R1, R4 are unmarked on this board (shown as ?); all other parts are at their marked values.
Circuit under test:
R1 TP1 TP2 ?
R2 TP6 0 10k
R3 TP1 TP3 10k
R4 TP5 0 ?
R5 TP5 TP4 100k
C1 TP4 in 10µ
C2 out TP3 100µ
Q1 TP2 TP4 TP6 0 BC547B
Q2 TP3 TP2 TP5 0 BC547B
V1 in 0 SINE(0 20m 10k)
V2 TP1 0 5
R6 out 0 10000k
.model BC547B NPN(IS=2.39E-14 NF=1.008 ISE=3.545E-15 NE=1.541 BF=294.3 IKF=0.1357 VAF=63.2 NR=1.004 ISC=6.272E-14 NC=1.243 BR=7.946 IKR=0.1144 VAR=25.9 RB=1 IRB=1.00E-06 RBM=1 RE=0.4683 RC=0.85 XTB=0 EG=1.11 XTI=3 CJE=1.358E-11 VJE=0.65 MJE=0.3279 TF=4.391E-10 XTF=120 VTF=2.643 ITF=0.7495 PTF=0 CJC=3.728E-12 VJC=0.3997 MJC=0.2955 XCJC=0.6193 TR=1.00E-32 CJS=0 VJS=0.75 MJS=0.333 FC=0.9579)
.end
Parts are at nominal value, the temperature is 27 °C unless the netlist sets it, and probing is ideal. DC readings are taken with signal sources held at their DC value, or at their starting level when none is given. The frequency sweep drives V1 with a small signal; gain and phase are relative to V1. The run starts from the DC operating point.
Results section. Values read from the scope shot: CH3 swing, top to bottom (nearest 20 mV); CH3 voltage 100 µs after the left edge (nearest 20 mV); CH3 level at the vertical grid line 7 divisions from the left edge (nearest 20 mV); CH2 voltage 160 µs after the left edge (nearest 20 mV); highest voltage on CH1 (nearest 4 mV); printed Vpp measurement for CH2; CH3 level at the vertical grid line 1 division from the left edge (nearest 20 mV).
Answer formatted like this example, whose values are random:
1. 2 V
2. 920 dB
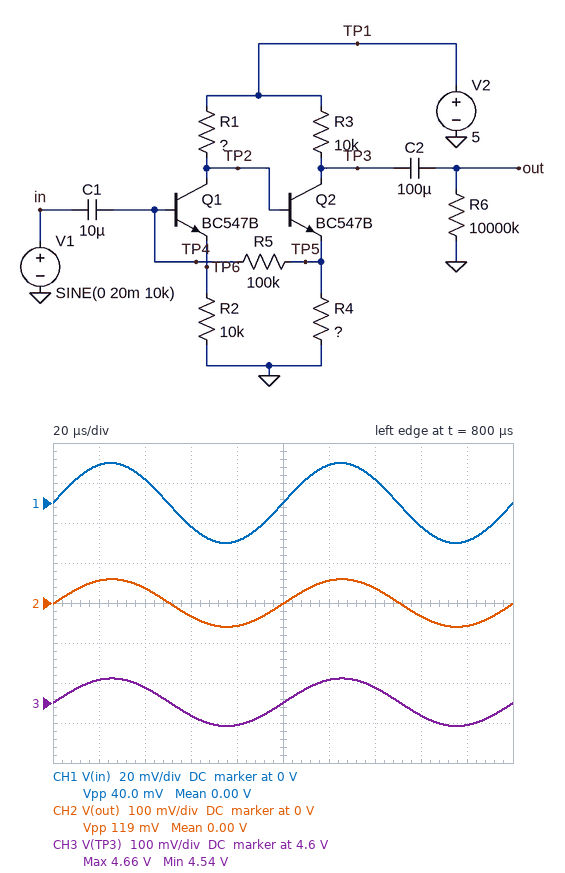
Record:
1. 120 mV
2. 4.60 V
3. 4.64 V
4. -40 mV
5. 20 mV
6. 119 mV
7. 4.66 V
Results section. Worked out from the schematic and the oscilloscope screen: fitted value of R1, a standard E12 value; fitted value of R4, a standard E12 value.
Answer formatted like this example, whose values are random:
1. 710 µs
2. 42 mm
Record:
1. 68 kΩ
2. 27 kΩ
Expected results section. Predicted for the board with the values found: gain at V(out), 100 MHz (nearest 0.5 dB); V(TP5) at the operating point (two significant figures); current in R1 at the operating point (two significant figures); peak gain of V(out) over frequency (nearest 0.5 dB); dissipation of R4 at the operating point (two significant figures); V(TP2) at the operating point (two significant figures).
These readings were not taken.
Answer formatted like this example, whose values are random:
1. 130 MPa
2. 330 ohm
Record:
1. 0 dB
2. 1.1 V
3. 50 µA
4. 9.5 dB
5. 43 µW
6. 1.6 V
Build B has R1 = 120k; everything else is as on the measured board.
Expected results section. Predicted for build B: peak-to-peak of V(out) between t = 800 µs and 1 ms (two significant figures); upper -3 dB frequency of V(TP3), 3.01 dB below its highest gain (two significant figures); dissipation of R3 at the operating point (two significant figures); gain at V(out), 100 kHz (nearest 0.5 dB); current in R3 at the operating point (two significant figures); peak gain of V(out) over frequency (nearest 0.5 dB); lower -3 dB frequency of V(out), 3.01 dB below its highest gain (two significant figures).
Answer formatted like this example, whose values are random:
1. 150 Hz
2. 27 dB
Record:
1. 200 mV
2. 200 kHz
3. 10 µW
4. 13.0 dB
5. 32 µA
6. 14.0 dB
7. 1.8 Hz
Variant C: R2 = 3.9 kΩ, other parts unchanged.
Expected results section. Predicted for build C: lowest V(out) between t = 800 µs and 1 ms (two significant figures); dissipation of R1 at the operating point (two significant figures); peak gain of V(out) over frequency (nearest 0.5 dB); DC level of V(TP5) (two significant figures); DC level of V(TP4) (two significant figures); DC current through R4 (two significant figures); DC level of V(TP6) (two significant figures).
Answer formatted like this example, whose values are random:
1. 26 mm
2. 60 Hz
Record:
1. -140 mV
2. 200 µW
3. 17.0 dB
4. 790 mV
5. 770 mV
6. 29 µA
7. 210 mV
